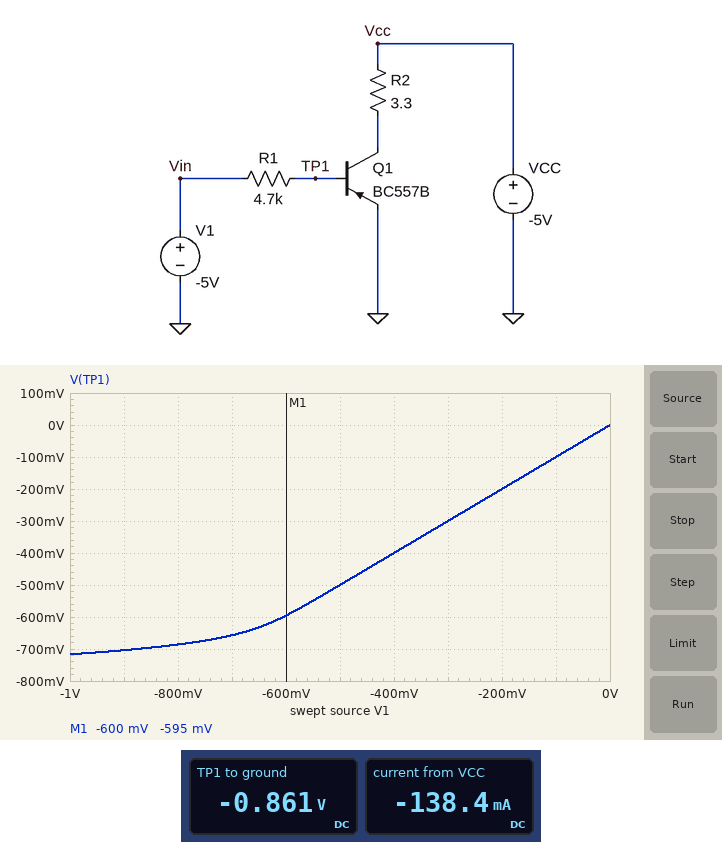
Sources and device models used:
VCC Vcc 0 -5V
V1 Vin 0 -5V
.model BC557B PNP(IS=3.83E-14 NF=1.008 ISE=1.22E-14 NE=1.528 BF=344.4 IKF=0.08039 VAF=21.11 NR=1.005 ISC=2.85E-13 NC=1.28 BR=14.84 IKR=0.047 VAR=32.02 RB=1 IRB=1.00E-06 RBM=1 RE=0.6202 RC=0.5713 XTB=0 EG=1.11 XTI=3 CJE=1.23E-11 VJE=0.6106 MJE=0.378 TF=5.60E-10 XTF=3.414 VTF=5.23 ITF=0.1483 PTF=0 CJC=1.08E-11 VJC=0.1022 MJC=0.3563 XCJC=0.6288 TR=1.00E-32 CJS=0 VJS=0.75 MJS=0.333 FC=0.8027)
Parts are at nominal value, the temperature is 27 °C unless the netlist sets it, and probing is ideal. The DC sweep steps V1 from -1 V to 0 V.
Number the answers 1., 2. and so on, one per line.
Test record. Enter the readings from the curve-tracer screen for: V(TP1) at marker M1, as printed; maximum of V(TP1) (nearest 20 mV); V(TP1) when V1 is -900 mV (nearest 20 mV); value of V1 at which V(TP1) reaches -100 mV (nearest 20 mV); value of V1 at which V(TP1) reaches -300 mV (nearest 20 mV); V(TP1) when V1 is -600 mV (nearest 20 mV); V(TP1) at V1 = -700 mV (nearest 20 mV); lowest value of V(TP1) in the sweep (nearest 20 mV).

1. -595 mV
2. 0 V
3. -700 mV
4. -100 mV
5. -300 mV
6. -600 mV
7. -660 mV
8. -720 mV
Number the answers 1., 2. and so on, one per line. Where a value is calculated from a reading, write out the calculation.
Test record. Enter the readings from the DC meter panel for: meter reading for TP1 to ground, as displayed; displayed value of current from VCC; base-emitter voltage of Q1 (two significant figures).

1. -0.861 V
2. -138.4 mA
3. -861 mV = -860 mV
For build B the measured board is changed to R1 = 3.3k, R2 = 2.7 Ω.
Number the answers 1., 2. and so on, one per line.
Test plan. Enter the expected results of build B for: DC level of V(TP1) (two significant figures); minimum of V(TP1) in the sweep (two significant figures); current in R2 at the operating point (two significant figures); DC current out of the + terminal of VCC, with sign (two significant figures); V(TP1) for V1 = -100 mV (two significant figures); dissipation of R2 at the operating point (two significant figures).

1. -890 mV
2. -730 mV
3. 170 mA
4. -170 mA
5. -100 mV
6. 79 mW
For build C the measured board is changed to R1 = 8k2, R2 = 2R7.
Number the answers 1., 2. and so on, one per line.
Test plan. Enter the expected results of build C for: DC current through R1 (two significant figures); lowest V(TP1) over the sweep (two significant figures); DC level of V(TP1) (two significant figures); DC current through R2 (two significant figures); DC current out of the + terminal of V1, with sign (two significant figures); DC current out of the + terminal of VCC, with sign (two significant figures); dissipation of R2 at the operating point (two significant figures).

1. 510 µA
2. -700 mV
3. -820 mV
4. 98 mA
5. -510 µA
6. -98 mA
7. 26 mW
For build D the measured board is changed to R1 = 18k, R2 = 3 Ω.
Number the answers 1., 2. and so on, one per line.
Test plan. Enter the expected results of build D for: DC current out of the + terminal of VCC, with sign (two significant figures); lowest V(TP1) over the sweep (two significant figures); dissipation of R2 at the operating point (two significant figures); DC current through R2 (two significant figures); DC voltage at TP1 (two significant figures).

1. -58 mA
2. -680 mV
3. 10 mW
4. 58 mA
5. -780 mV
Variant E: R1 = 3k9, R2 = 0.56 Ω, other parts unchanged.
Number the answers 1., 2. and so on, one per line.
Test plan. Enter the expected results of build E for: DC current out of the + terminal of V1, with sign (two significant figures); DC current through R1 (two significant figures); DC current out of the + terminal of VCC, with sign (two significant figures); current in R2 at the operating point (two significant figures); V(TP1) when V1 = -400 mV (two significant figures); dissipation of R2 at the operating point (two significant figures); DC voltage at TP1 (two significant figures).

1. -1.1 mA
2. 1.1 mA
3. -160 mA
4. 160 mA
5. -400 mV
6. 14 mW
7. -880 mV
